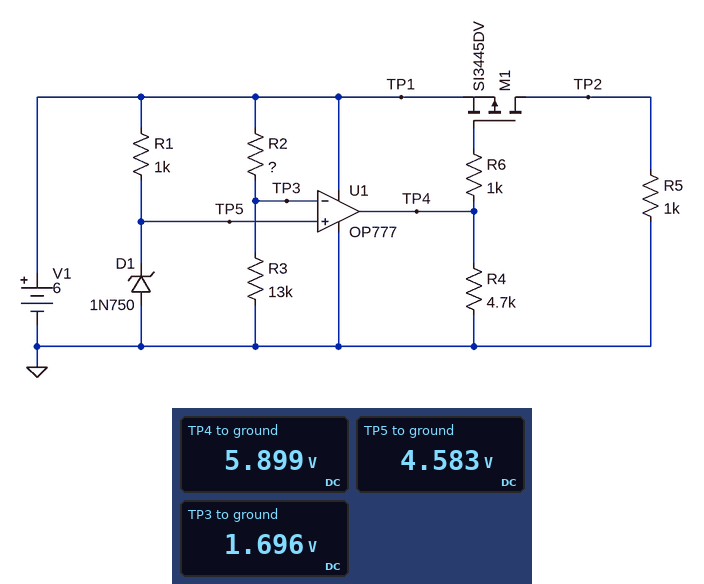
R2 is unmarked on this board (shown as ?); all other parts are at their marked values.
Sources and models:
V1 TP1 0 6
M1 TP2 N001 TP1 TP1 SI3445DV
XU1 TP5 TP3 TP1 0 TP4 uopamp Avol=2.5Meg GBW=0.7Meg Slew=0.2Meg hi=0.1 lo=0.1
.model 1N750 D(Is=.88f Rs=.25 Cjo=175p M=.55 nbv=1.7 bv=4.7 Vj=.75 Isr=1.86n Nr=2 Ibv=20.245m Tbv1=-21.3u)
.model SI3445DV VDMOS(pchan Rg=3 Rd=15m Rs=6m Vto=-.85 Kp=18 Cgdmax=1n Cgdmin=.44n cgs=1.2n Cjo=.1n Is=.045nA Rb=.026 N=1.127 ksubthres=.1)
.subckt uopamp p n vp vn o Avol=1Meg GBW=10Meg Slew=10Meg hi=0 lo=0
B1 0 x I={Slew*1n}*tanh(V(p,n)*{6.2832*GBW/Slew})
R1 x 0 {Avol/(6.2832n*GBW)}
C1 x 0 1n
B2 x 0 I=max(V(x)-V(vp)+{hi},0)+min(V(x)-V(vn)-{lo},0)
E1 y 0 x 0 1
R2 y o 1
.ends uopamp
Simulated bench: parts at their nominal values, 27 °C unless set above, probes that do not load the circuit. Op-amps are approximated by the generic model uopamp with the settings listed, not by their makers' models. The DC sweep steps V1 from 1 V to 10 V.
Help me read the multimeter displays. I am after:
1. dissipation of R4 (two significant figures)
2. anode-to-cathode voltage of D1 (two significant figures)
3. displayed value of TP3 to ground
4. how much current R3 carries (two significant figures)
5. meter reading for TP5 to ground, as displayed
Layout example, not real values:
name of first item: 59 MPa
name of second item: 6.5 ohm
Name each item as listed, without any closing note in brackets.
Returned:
dissipation of R4: 7.4 mW
anode-to-cathode voltage of D1: -4.6 V
displayed value of TP3 to ground: 1.696 V
how much current R3 carries: 130 µA
meter reading for TP5 to ground, as displayed: 4.583 V
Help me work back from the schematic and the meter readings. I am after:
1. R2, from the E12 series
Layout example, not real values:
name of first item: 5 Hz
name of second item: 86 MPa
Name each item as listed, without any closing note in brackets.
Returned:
R2, from the E12 series: 33 kΩ
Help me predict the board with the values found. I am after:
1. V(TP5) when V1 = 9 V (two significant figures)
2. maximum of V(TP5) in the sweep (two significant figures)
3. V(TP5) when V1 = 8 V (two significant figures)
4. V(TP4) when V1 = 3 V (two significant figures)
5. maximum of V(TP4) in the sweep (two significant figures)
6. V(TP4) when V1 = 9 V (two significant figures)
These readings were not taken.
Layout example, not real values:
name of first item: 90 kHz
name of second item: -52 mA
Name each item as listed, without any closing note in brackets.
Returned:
V(TP5) when V1 = 9 V: 4.6 V
maximum of V(TP5) in the sweep: 4.6 V
V(TP5) when V1 = 8 V: 4.6 V
V(TP4) when V1 = 3 V: 2.9 V
maximum of V(TP4) in the sweep: 9.9 V
V(TP4) when V1 = 9 V: 8.9 V
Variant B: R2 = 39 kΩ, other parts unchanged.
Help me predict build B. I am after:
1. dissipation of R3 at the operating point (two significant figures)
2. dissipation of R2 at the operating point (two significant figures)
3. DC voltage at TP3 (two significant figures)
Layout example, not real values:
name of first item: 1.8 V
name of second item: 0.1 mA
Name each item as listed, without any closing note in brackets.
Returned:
dissipation of R3 at the operating point: 170 µW
dissipation of R2 at the operating point: 520 µW
DC voltage at TP3: 1.5 V
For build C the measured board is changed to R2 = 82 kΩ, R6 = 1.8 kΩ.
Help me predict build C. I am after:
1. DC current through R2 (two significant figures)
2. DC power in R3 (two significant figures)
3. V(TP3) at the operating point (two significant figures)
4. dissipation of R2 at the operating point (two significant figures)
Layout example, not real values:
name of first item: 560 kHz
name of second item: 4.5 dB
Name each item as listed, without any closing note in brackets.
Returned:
DC current through R2: 63 µA
DC power in R3: 52 µW
V(TP3) at the operating point: 820 mV
dissipation of R2 at the operating point: 330 µW
